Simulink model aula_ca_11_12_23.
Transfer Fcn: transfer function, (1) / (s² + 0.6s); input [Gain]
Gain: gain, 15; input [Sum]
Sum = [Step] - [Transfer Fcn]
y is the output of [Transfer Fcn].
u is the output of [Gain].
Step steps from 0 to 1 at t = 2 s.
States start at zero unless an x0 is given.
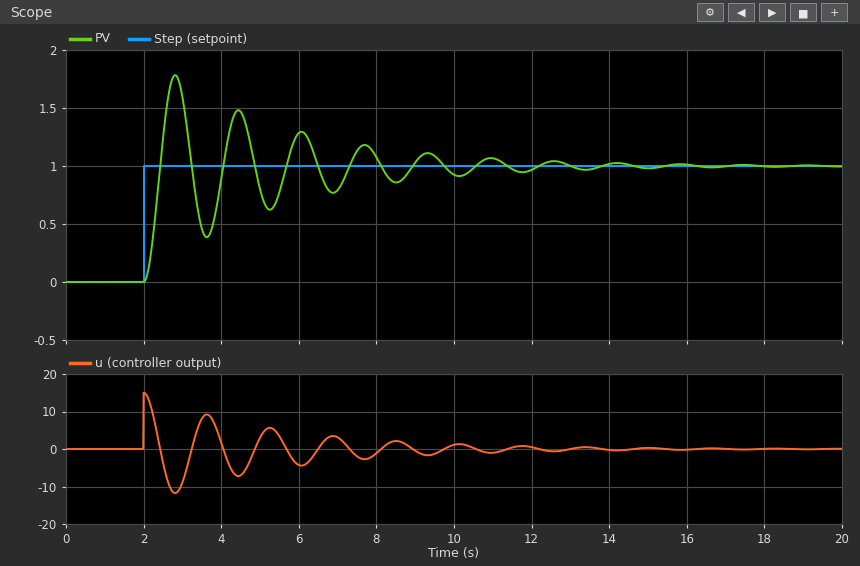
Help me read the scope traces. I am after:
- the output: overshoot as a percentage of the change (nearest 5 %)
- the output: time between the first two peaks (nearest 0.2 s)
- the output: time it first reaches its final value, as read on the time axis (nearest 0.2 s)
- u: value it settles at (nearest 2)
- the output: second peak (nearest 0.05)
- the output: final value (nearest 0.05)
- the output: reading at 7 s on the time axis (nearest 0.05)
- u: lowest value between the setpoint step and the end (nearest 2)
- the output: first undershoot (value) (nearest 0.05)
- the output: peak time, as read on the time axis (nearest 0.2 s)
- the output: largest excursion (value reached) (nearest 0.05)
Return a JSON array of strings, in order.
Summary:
["80 %", "1.6 s", "2.4 s", "0", "1.50", "1.00", "0.80", "-12", "0.40", "2.8 s", "1.80"]
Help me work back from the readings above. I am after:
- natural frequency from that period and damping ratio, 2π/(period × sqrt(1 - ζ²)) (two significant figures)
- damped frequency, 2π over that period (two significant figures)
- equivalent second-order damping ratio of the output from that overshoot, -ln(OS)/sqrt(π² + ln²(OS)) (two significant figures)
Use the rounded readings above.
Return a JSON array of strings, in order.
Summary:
["3.9 rad/s", "3.9 rad/s", "0.071"]
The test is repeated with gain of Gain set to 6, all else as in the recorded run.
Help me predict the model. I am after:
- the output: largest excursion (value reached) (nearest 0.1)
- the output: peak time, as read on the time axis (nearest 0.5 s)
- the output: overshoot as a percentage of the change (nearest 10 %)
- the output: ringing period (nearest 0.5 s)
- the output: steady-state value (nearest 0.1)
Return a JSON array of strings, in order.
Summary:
["1.7", "3.5 s", "70 %", "2.5 s", "1.0"]
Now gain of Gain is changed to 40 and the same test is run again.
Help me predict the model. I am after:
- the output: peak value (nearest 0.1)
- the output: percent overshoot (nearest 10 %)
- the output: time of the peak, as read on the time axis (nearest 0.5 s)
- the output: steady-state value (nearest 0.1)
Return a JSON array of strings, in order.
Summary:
["1.9", "90 %", "2.5 s", "1.0"]
